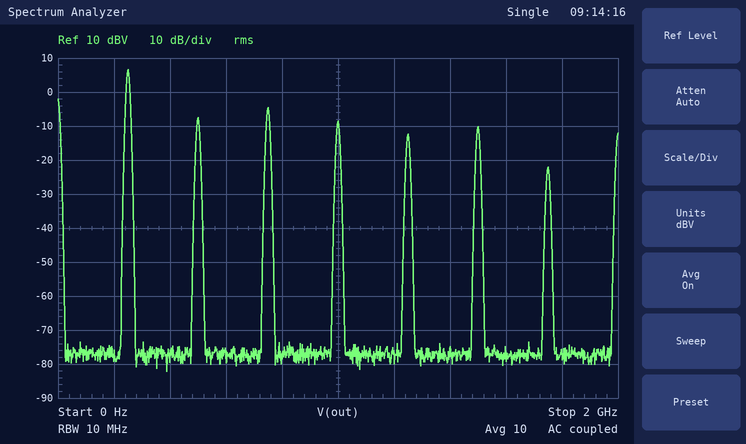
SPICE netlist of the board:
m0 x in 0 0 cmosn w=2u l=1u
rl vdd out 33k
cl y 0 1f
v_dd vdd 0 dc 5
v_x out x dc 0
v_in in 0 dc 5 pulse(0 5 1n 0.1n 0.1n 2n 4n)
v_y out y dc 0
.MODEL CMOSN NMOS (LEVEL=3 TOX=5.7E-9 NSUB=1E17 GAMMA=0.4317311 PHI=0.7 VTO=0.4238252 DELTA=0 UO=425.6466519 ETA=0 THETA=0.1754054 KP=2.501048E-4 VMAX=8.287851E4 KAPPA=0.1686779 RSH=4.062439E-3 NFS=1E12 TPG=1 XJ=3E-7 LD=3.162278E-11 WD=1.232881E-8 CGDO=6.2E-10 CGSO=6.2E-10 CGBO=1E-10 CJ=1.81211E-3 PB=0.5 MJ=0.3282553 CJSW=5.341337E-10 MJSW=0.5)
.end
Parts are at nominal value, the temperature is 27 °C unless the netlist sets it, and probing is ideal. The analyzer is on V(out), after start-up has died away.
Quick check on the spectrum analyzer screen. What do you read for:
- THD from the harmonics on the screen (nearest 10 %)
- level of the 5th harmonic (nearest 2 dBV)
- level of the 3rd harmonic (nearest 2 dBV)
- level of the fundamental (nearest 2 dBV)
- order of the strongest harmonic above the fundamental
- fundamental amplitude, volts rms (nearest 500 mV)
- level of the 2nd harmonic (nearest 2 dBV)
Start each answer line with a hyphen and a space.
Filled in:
- 40 %
- -12 dBV
- -4 dBV
- 6 dBV
- 3
- 2.0 V
- -8 dBV
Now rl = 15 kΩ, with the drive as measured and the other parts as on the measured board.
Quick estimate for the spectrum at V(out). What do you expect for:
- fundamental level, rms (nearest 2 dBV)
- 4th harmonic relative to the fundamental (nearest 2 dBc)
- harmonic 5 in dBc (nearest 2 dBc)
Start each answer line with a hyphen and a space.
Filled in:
- 6 dBV
- -18 dBc
- -16 dBc
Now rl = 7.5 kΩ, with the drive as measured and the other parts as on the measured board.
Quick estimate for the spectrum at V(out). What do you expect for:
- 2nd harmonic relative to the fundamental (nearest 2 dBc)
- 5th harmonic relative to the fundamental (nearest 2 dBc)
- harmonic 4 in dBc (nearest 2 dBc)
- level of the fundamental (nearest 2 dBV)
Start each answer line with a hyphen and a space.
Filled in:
- -20 dBc
- -16 dBc
- -20 dBc
- 6 dBV
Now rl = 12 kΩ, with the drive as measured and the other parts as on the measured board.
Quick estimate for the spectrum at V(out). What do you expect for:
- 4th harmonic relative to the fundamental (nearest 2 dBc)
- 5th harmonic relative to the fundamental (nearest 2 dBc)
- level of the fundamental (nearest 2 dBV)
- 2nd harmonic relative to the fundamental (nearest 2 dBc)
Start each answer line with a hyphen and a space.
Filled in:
- -18 dBc
- -16 dBc
- 6 dBV
- -18 dBc
